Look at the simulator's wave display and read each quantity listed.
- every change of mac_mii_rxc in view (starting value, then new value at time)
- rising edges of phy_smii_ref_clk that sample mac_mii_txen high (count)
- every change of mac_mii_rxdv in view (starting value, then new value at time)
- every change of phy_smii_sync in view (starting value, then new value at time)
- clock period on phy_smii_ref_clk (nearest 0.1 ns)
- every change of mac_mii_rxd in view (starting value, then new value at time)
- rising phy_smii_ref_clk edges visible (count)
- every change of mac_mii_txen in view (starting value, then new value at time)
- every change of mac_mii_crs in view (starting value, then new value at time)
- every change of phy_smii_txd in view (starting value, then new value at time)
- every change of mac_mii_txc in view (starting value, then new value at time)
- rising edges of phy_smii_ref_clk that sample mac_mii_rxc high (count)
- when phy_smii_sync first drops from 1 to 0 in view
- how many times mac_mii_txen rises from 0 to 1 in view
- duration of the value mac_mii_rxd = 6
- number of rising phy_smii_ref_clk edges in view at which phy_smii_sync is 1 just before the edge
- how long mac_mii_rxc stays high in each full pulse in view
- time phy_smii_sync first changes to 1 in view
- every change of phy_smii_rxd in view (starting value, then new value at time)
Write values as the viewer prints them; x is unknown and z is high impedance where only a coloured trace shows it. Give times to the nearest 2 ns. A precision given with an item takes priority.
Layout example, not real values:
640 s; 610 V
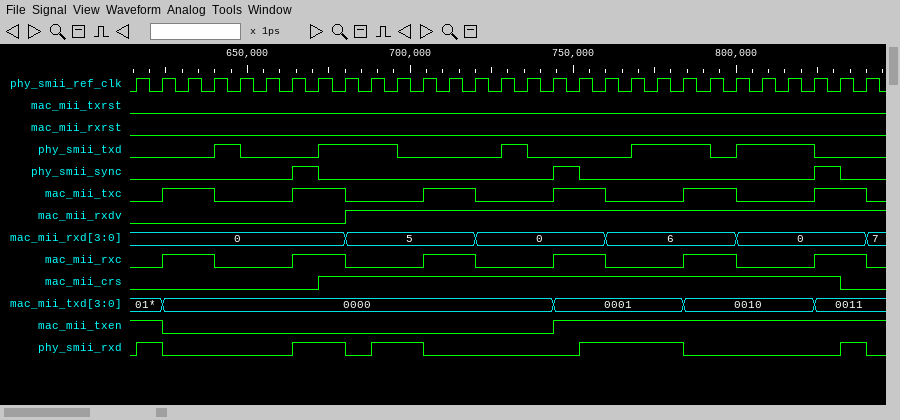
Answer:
0, 1 at 624 ns, 0 at 640 ns, 1 at 664 ns, 0 at 680 ns, 1 at 704 ns, 0 at 720 ns, 1 at 744 ns, 0 at 760 ns, 1 at 784 ns, 0 at 800 ns, 1 at 824 ns, 0 at 840 ns; 14; 0, 1 at 680 ns; 0, 1 at 664 ns, 0 at 672 ns, 1 at 744 ns, 0 at 752 ns, 1 at 824 ns, 0 at 832 ns; 8 ns; 0, 5 at 680 ns, 0 at 720 ns, 6 at 760 ns, 0 at 800 ns, 7 at 840 ns; 29; 1, 0 at 624 ns, 1 at 744 ns; 0, 1 at 672 ns, 0 at 832 ns; 0, 1 at 640 ns, 0 at 648 ns, 1 at 672 ns, 0 at 696 ns, 1 at 728 ns, 0 at 736 ns, 1 at 768 ns, 0 at 792 ns, 1 at 800 ns, 0 at 824 ns; 0, 1 at 624 ns, 0 at 640 ns, 1 at 664 ns, 0 at 680 ns, 1 at 704 ns, 0 at 720 ns, 1 at 744 ns, 0 at 760 ns, 1 at 784 ns, 0 at 800 ns, 1 at 824 ns, 0 at 840 ns; 12; 672 ns; 1; 40 ns; 3; 16 ns, 16 ns, 16 ns, 16 ns, 16 ns, 16 ns; 664 ns; 0, 1 at 616 ns, 0 at 624 ns, 1 at 664 ns, 0 at 680 ns, 1 at 688 ns, 0 at 704 ns, 1 at 752 ns, 0 at 784 ns, 1 at 832 ns, 0 at 840 ns
